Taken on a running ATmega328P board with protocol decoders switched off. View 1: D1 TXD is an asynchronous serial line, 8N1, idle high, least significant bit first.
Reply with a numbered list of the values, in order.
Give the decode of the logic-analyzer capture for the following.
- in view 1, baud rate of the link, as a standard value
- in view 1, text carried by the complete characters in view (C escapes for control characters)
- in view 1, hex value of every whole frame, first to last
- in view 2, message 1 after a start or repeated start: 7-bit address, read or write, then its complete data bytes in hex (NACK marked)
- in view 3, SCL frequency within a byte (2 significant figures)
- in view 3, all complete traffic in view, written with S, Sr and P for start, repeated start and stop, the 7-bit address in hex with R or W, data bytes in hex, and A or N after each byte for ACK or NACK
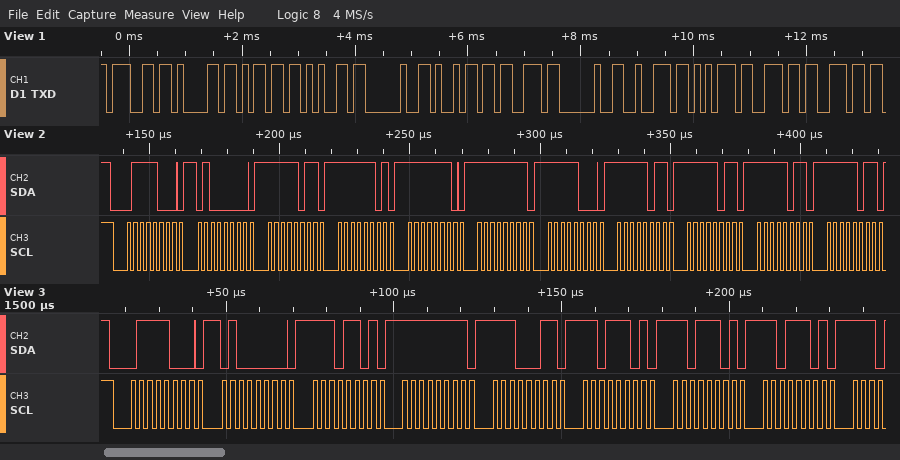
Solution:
1. 9600 baud
2. "game is runn"
3. 67 61 6D 65 20 69 73 20 72 75 6E 6E
4. 0x3C write: 40 FB FD FE FF F8 FB FB FB FB
5. 400 kHz
6. S 3CW A 40 A ED A FF A E3 A DD A DD A DD A
